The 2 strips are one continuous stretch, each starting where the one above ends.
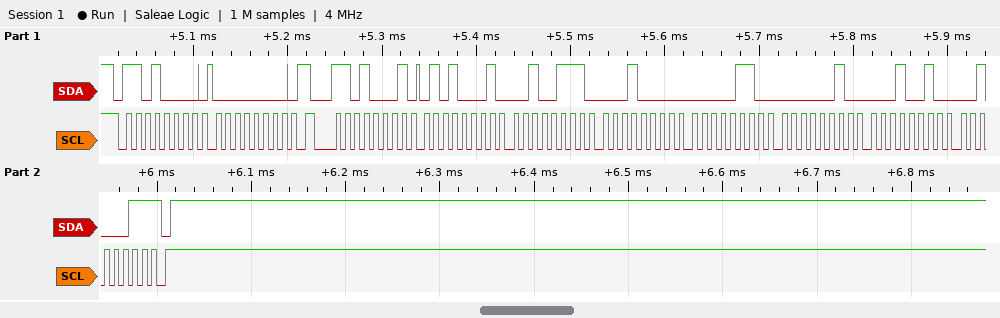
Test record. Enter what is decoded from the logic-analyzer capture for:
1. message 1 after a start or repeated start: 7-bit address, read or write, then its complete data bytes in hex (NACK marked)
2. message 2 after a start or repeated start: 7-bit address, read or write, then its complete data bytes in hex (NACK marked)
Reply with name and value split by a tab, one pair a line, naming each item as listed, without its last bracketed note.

message 1 after a start or repeated start: 7-bit address, read or write, then its complete data bytes in hex	0x68 write: 00
message 2 after a start or repeated start: 7-bit address, read or write, then its complete data bytes in hex	0x68 read: 51 27 10 06 02 12 23 NACK
